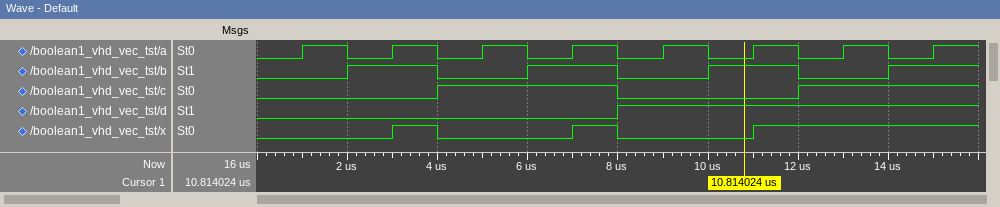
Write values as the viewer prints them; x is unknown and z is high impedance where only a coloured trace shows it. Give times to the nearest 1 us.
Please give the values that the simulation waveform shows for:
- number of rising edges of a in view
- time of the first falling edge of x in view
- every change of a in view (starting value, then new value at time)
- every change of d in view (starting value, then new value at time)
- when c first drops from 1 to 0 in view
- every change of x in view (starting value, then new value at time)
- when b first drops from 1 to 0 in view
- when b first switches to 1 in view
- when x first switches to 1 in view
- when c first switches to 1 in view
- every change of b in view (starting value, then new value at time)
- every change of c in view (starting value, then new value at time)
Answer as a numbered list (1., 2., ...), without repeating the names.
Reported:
1. 8
2. 4 us
3. 0, 1 at 1 us, 0 at 2 us, 1 at 3 us, 0 at 4 us, 1 at 5 us, 0 at 6 us, 1 at 7 us, 0 at 8 us, 1 at 9 us, 0 at 10 us, 1 at 11 us, 0 at 12 us, 1 at 13 us, 0 at 14 us, 1 at 15 us
4. 0, 1 at 8 us
5. 8 us
6. 0, 1 at 3 us, 0 at 4 us, 1 at 7 us, 0 at 8 us, 1 at 11 us
7. 4 us
8. 2 us
9. 3 us
10. 4 us
11. 0, 1 at 2 us, 0 at 4 us, 1 at 6 us, 0 at 8 us, 1 at 10 us, 0 at 12 us, 1 at 14 us
12. 0, 1 at 4 us, 0 at 8 us, 1 at 12 us
